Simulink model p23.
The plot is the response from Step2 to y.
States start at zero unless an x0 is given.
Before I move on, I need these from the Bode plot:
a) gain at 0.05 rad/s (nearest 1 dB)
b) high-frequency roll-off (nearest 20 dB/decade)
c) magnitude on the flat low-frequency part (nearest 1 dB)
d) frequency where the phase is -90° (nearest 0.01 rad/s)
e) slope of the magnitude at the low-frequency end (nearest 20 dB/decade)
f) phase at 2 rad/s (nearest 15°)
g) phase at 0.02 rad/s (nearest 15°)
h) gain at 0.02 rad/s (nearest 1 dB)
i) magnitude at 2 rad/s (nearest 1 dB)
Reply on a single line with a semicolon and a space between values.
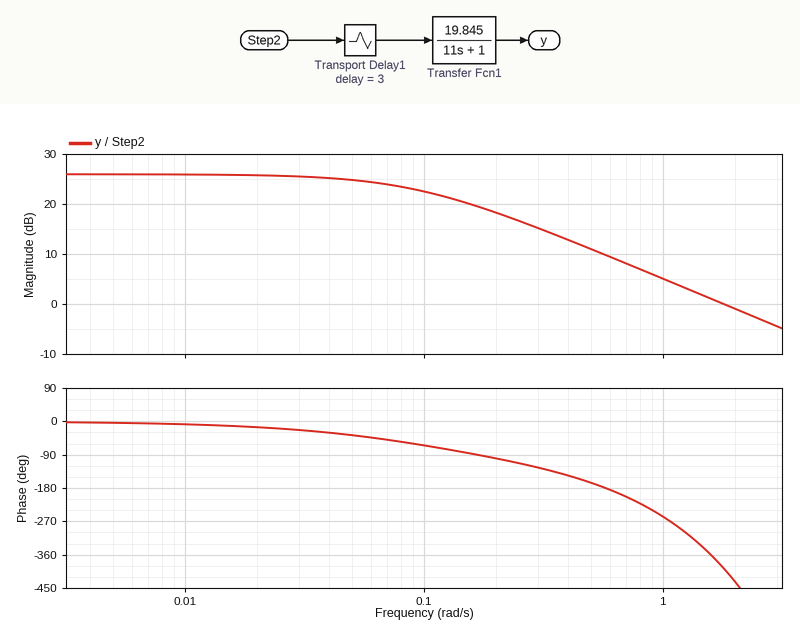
25 dB; -20 dB/decade; 26 dB; 0.17 rad/s; 0 dB/decade; -435°; -15°; 26 dB; -1 dB
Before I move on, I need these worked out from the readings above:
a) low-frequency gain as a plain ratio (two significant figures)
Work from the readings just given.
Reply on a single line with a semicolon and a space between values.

20
